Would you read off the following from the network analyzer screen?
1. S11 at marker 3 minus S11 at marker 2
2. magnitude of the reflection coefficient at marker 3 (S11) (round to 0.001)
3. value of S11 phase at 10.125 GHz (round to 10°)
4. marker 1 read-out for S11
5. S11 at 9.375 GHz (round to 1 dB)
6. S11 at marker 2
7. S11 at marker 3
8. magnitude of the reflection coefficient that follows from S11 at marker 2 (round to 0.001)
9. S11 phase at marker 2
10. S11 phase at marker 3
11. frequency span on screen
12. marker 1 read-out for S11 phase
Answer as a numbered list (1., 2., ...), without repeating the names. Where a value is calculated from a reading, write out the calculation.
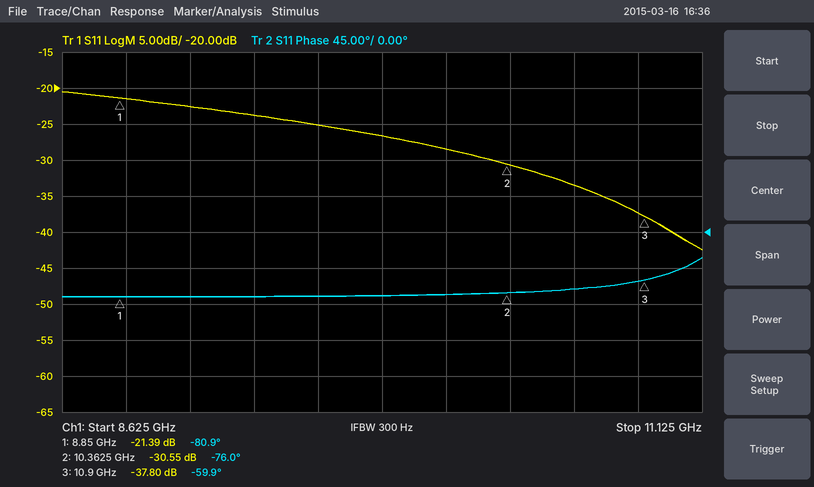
1. -37.8 − (-30.55) = -7.25 dB
2. 10^(-37.8/20) ≈ 0.013
3. -80°
4. -21.39 dB
5. -24 dB
6. -30.55 dB
7. -37.80 dB
8. 10^(-30.55/20) ≈ 0.030
9. -76.0°
10. -59.9°
11. 2.5 GHz
12. -80.9°
